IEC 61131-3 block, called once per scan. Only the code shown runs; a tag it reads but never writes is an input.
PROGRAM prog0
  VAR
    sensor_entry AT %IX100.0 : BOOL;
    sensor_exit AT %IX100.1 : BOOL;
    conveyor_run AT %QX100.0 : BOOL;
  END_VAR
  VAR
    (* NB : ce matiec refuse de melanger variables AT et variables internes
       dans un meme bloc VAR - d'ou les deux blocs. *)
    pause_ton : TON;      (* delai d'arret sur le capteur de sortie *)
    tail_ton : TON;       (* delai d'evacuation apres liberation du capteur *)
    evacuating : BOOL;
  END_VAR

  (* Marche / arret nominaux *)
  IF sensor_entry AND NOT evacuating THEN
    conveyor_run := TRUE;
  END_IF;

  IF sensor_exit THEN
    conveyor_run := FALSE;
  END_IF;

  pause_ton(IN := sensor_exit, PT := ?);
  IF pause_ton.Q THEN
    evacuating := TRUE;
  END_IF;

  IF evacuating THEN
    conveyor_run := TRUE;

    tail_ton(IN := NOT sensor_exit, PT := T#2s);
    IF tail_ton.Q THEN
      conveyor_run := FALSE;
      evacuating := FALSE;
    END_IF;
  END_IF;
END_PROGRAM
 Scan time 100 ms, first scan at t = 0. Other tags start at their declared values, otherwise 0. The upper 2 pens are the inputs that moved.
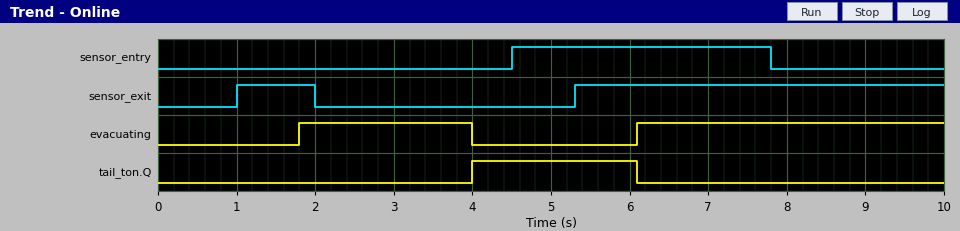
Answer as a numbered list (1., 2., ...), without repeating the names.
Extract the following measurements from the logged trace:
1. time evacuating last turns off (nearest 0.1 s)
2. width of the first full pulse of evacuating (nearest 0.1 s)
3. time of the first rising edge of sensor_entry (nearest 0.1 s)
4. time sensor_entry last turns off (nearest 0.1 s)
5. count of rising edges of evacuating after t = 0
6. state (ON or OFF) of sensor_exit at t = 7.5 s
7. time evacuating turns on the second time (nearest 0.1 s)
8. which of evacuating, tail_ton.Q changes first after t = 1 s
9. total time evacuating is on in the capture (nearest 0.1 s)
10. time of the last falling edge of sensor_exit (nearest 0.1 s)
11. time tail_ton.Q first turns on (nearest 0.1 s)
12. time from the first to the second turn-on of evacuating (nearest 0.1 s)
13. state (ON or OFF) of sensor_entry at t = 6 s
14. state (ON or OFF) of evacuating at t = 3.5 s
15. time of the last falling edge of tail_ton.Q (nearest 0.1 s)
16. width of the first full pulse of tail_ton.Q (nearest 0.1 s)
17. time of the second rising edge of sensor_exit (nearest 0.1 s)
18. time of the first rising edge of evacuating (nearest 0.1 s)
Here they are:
1. 4.0 s
2. 2.2 s
3. 4.5 s
4. 7.8 s
5. 2
6. ON
7. 6.1 s
8. evacuating
9. 6.1 s
10. 2.0 s
11. 4.0 s
12. 4.3 s
13. ON
14. ON
15. 6.1 s
16. 2.1 s
17. 5.3 s
18. 1.8 s
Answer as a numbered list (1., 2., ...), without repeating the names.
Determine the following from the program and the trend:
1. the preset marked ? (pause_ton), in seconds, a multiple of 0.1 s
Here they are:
1. 0.8 s
